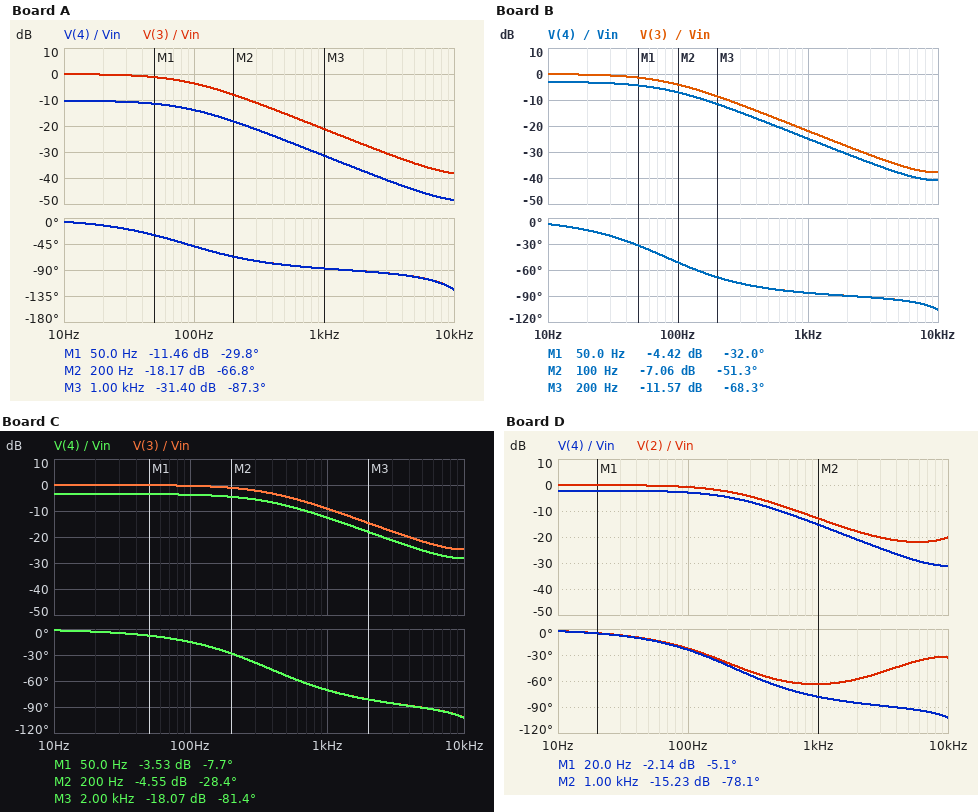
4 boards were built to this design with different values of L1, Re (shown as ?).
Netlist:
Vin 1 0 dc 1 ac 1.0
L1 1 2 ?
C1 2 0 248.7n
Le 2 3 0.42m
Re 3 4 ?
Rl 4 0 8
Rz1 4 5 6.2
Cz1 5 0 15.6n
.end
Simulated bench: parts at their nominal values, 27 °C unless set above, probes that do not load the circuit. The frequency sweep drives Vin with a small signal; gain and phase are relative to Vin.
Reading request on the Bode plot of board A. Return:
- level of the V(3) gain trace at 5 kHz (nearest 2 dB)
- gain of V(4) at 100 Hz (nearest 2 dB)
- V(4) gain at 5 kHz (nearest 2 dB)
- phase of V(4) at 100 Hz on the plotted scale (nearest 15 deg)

-34 dB
-14 dB
-44 dB
-45 deg
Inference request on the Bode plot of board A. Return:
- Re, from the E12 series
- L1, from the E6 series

18 Ω
47 mH
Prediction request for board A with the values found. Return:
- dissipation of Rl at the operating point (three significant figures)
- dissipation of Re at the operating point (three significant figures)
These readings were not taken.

11.8 mW
26.6 mW
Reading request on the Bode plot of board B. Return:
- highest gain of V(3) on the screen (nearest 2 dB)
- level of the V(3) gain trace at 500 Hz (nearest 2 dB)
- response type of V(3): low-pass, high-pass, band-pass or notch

0 dB
-16 dB
low-pass
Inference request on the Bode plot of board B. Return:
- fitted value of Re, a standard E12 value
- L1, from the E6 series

3.3 Ω
22 mH
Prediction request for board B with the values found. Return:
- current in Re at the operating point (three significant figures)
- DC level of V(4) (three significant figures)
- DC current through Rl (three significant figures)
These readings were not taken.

88.5 mA
708 mV
88.5 mA
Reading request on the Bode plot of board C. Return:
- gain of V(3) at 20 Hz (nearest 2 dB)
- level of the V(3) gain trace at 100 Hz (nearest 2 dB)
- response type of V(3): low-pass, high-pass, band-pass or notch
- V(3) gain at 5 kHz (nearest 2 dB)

0 dB
0 dB
low-pass
-22 dB
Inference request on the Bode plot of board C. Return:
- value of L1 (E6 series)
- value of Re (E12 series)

4.7 mH
3.9 Ω
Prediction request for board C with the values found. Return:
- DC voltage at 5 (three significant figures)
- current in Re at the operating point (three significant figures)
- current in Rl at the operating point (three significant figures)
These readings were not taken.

672 mV
84.0 mA
84.0 mA
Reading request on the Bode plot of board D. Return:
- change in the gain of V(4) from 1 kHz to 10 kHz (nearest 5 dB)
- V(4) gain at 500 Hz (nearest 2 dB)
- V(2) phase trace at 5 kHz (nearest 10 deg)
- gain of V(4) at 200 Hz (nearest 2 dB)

-15 dB
-10 dB
-40 deg
-4 dB
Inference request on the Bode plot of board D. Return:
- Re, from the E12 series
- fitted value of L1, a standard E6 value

2.2 Ω
6.8 mH
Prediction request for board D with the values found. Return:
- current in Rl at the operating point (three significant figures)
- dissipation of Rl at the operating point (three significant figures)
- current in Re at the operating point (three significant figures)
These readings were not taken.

98.0 mA
76.9 mW
98.0 mA
